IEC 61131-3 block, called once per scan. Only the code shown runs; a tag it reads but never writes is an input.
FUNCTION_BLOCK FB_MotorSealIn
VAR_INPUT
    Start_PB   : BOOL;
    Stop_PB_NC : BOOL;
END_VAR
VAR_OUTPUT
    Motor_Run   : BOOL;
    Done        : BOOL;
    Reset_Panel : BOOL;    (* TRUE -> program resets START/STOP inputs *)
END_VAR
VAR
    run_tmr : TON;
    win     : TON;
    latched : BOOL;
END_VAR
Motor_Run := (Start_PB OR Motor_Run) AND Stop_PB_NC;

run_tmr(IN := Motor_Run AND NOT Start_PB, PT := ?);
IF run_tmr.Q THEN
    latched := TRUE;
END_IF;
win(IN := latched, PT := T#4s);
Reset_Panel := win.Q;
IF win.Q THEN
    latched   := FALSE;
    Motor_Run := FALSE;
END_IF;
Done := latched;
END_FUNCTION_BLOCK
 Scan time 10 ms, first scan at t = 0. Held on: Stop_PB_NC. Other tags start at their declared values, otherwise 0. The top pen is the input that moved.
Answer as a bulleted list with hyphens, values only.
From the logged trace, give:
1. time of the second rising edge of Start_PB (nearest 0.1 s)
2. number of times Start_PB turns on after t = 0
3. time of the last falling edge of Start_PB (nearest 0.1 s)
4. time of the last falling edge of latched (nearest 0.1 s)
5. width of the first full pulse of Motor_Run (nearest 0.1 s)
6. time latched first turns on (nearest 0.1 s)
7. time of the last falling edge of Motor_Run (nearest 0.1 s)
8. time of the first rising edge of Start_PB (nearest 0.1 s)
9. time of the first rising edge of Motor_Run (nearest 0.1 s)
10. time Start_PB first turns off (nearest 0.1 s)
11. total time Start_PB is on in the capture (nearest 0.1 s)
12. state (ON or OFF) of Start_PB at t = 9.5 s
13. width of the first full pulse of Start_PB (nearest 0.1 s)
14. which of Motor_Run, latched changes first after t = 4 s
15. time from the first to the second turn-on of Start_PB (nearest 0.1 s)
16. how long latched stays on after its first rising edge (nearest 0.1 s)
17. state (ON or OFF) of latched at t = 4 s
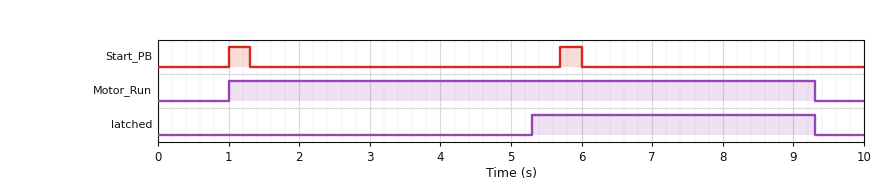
- 5.7 s
- 2
- 6.0 s
- 9.3 s
- 8.3 s
- 5.3 s
- 9.3 s
- 1.0 s
- 1.0 s
- 1.3 s
- 0.6 s
- OFF
- 0.3 s
- latched
- 4.7 s
- 4.0 s
- OFF
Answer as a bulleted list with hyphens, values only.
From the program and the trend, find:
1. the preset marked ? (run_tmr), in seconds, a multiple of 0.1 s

- 4.0 s
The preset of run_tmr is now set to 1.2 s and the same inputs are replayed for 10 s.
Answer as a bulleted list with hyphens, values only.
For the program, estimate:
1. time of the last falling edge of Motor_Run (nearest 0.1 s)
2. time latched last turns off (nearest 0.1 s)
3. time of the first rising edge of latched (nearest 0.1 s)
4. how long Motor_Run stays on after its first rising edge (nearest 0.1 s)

- 6.5 s
- 6.5 s
- 2.5 s
- 5.5 s
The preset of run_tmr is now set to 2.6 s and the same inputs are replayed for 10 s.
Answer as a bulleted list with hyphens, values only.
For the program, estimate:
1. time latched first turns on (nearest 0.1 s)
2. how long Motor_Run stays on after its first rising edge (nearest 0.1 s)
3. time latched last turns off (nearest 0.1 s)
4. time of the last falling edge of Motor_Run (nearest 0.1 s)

- 3.9 s
- 6.9 s
- 7.9 s
- 7.9 s
